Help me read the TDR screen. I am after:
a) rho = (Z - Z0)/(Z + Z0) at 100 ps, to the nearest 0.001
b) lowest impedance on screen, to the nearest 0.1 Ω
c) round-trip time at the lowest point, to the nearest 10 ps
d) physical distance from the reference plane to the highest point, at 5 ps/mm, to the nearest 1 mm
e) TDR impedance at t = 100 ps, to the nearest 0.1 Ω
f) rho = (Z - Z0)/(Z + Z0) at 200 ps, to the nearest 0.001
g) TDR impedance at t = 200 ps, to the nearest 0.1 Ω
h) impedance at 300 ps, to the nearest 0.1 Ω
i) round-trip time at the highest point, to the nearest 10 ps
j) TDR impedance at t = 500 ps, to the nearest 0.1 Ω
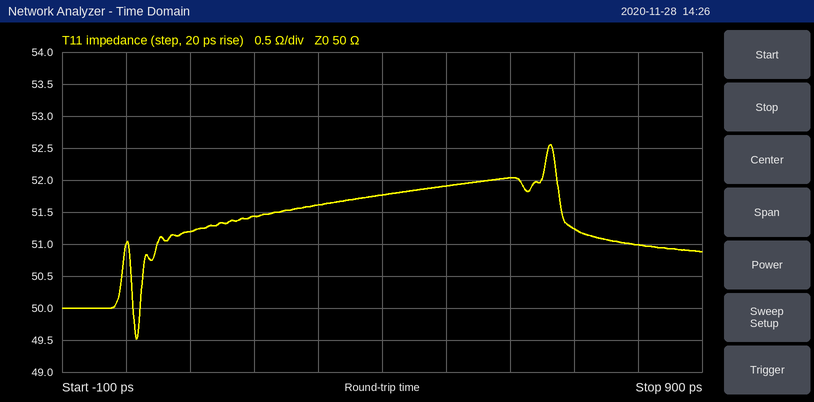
+0.012
49.5 Ω
20 ps
66 mm
51.2 Ω
+0.014
51.4 Ω
51.6 Ω
660 ps
51.9 Ω
